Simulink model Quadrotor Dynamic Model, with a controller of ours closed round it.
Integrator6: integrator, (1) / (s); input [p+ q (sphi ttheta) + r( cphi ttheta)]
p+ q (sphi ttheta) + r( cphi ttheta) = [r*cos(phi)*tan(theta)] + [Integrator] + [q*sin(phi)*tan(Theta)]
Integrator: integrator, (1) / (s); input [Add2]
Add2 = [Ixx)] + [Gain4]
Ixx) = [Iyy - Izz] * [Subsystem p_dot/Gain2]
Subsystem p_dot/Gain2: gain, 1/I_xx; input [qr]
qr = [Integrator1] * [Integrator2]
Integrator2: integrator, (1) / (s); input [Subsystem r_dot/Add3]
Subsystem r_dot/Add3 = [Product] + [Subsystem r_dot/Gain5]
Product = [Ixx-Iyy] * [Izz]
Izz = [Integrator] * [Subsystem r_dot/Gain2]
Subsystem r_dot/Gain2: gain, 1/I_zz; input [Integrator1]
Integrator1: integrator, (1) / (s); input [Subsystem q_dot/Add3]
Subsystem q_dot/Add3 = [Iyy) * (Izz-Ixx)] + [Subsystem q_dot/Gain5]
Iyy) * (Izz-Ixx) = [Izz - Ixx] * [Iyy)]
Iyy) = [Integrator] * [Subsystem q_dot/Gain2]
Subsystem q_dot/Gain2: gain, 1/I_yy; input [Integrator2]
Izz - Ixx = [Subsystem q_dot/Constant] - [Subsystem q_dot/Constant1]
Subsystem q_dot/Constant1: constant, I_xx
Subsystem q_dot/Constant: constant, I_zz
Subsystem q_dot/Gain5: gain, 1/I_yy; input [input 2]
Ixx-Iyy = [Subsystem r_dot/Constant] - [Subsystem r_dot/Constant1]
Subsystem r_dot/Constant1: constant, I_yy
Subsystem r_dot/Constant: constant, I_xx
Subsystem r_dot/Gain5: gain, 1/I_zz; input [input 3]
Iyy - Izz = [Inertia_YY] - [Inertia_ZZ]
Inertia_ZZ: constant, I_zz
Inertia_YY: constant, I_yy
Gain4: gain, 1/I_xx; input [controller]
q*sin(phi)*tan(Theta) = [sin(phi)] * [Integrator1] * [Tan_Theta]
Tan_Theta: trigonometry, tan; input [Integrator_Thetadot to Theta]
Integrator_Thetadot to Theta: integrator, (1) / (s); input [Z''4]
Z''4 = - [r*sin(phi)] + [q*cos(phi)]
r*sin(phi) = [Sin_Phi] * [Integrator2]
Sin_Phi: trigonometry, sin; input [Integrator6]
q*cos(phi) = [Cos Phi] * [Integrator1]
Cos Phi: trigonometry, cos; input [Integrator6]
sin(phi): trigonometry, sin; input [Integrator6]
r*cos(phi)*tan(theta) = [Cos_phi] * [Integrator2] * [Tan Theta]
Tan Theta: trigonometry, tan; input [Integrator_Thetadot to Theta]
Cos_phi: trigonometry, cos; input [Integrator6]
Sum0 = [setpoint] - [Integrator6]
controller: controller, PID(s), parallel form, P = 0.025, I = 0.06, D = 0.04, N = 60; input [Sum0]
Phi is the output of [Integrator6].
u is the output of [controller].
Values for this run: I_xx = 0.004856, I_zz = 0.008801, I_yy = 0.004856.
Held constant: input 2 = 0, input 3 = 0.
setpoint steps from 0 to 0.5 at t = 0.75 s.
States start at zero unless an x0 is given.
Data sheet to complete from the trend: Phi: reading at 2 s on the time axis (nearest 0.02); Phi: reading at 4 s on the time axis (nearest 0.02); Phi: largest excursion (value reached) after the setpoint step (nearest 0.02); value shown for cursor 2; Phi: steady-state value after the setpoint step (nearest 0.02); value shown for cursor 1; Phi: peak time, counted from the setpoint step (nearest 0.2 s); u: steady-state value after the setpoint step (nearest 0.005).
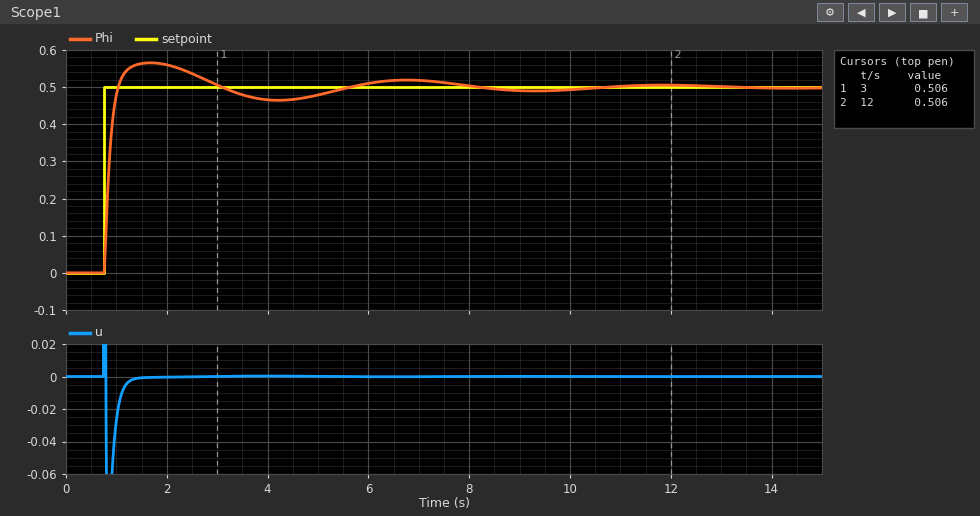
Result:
0.56
0.46
0.56
0.506
0.50
0.506
1.0 s
0.000
